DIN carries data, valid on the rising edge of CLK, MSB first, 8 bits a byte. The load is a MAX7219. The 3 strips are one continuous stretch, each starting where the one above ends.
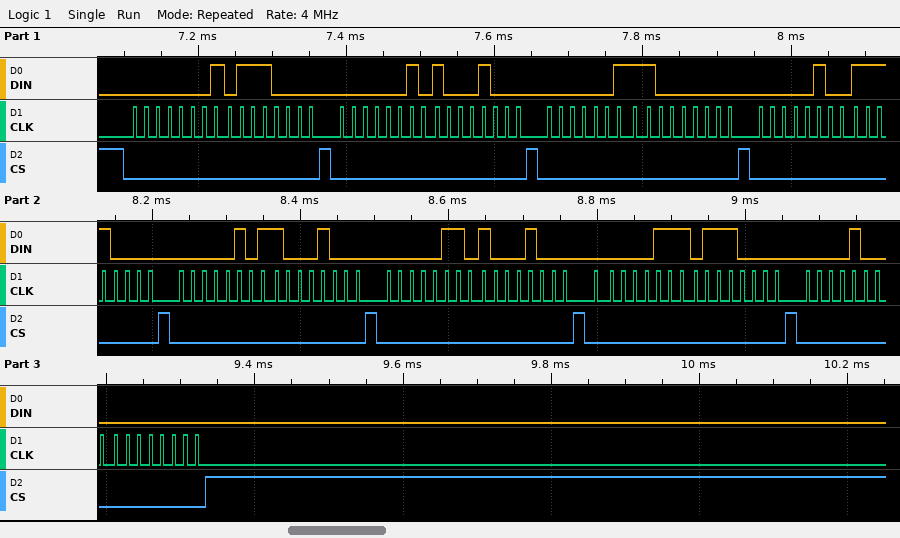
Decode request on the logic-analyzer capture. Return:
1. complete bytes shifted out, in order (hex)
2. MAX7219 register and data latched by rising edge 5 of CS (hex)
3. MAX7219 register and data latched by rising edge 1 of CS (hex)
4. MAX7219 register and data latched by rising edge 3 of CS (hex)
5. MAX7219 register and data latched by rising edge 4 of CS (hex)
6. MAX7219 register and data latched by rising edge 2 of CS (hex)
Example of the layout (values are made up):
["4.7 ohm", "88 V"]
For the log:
["01 70 02 88 03 80 04 F0 05 88 06 88 07 70 08 00", "register 0x5, data 0x88", "register 0x1, data 0x70", "register 0x3, data 0x80", "register 0x4, data 0xF0", "register 0x2, data 0x88"]
